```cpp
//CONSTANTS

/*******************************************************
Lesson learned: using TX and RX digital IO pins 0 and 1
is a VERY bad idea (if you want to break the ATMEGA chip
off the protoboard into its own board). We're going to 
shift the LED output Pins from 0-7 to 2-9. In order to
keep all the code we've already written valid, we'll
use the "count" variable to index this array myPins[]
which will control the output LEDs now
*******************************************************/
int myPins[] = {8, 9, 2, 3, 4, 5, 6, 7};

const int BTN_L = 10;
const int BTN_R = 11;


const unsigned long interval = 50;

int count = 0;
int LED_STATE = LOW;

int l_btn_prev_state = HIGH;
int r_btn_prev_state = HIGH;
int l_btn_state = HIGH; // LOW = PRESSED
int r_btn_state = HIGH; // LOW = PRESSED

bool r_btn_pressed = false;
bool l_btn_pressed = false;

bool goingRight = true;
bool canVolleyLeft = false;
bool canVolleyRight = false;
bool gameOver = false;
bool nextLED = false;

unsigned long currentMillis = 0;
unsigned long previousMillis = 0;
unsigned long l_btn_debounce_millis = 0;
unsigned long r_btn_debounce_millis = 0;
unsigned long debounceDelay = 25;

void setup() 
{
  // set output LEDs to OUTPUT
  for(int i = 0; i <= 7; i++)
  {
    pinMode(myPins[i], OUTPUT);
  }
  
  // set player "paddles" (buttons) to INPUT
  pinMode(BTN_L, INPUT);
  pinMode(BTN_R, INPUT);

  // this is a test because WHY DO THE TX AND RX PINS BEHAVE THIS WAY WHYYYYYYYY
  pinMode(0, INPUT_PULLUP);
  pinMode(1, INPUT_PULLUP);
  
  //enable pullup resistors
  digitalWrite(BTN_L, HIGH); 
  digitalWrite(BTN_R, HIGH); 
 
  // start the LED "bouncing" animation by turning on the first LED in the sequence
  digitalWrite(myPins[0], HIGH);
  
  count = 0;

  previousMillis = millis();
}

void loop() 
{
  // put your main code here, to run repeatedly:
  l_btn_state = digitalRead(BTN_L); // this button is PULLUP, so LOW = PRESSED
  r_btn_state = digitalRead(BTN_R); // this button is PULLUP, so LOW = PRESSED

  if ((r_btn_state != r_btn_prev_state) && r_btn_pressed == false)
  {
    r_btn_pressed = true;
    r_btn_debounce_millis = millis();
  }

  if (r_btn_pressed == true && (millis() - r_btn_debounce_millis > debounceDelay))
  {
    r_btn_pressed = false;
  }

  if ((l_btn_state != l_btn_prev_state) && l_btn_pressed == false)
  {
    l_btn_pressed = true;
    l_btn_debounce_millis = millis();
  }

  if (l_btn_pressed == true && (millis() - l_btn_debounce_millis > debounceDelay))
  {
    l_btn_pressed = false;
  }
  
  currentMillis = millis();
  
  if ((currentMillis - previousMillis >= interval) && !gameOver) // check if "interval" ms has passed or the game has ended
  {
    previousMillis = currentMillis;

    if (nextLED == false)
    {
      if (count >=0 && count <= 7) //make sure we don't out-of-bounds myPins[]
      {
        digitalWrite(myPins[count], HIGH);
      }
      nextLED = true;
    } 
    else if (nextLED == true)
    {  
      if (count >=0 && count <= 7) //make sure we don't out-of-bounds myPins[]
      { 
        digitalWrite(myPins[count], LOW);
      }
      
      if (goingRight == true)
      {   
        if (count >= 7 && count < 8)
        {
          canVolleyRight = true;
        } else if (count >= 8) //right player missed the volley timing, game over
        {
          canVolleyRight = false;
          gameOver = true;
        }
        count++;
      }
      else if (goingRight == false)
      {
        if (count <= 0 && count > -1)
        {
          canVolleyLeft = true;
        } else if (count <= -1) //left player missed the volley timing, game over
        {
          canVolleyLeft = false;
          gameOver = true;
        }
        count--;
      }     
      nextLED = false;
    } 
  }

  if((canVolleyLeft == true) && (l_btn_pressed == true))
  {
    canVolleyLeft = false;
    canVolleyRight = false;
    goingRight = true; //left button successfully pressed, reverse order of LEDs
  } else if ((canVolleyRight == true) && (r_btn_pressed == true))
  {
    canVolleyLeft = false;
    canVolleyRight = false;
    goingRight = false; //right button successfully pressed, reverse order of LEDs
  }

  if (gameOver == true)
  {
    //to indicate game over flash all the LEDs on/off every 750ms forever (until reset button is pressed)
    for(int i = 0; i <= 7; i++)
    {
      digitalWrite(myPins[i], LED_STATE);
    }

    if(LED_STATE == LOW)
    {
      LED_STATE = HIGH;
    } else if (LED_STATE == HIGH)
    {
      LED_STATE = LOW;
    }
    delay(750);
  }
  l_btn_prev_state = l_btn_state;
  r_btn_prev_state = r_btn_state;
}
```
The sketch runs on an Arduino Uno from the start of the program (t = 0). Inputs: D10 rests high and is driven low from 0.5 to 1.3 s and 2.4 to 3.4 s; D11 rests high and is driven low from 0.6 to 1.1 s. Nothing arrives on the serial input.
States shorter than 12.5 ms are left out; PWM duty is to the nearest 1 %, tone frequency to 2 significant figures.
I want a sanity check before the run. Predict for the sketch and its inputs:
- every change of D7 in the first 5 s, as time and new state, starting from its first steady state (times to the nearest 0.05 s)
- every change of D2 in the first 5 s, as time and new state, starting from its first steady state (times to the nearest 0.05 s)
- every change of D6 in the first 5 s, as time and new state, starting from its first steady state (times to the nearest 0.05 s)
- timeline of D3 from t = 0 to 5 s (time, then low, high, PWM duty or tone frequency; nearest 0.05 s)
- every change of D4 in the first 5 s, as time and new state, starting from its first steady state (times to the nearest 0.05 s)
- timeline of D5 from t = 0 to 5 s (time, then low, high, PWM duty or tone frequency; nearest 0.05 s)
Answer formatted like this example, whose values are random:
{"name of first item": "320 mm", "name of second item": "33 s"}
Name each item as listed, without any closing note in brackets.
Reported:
{"every change of D7 in the first 5 s, as time and new state, starting from its first steady state": "0 s low; 0.75 s high; 0.8 s low; 1.65 s high; 2.4 s low; 3.15 s high; 3.9 s low; 4.65 s high", "every change of D2 in the first 5 s, as time and new state, starting from its first steady state": "0 s low; 0.25 s high; 0.3 s low; 1.65 s high; 2.4 s low; 3.15 s high; 3.9 s low; 4.65 s high", "every change of D6 in the first 5 s, as time and new state, starting from its first steady state": "0 s low; 0.65 s high; 0.7 s low; 1.65 s high; 2.4 s low; 3.15 s high; 3.9 s low; 4.65 s high", "timeline of D3 from t = 0 to 5 s": "0 s low; 0.35 s high; 0.4 s low; 1.65 s high; 2.4 s low; 3.15 s high; 3.9 s low; 4.65 s high", "every change of D4 in the first 5 s, as time and new state, starting from its first steady state": "0 s low; 0.45 s high; 0.5 s low; 1.65 s high; 2.4 s low; 3.15 s high; 3.9 s low; 4.65 s high", "timeline of D5 from t = 0 to 5 s": "0 s low; 0.55 s high; 0.6 s low; 1.65 s high; 2.4 s low; 3.15 s high; 3.9 s low; 4.65 s high"}
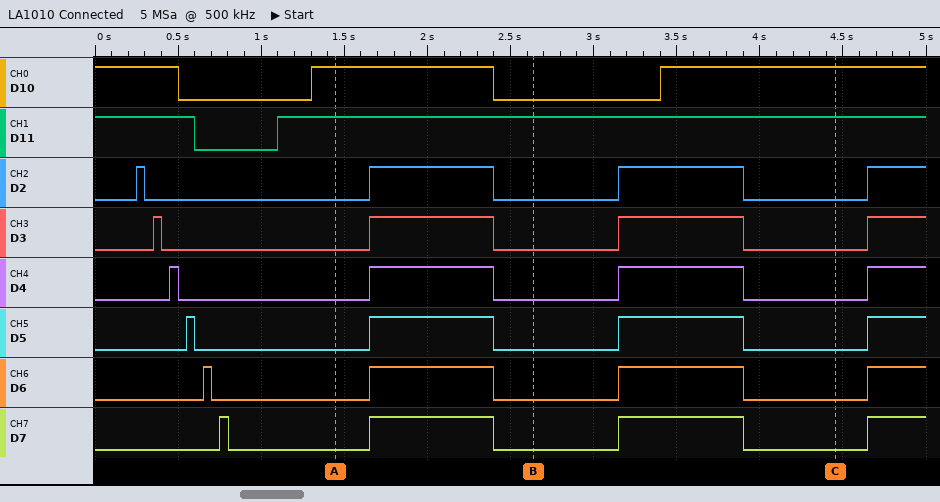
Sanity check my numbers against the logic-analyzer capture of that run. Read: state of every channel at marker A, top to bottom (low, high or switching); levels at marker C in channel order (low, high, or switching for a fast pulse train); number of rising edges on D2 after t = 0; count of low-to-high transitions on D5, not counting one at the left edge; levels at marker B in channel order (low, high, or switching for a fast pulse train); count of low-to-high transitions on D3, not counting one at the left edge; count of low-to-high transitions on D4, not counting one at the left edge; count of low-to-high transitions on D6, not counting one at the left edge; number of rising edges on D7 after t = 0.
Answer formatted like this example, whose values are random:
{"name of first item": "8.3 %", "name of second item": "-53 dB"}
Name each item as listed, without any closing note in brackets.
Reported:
{"state of every channel at marker A, top to bottom": "D10 high, D11 high, D2 low, D3 low, D4 low, D5 low, D6 low, D7 low", "levels at marker C in channel order": "D10 high, D11 high, D2 low, D3 low, D4 low, D5 low, D6 low, D7 low", "number of rising edges on D2 after t = 0": "4", "count of low-to-high transitions on D5, not counting one at the left edge": "4", "levels at marker B in channel order": "D10 low, D11 high, D2 low, D3 low, D4 low, D5 low, D6 low, D7 low", "count of low-to-high transitions on D3, not counting one at the left edge": "4", "count of low-to-high transitions on D4, not counting one at the left edge": "4", "count of low-to-high transitions on D6, not counting one at the left edge": "4", "number of rising edges on D7 after t = 0": "4"}
